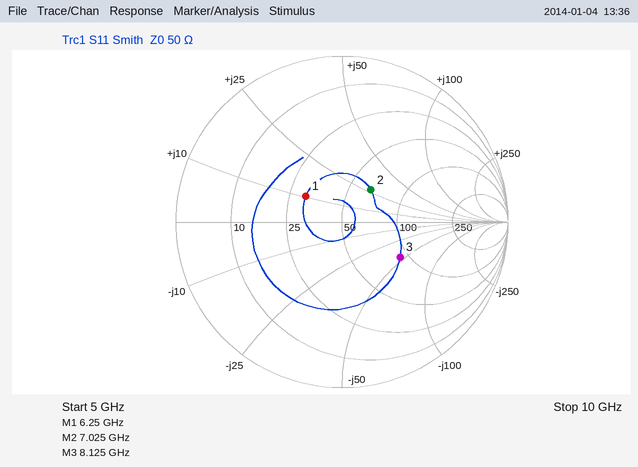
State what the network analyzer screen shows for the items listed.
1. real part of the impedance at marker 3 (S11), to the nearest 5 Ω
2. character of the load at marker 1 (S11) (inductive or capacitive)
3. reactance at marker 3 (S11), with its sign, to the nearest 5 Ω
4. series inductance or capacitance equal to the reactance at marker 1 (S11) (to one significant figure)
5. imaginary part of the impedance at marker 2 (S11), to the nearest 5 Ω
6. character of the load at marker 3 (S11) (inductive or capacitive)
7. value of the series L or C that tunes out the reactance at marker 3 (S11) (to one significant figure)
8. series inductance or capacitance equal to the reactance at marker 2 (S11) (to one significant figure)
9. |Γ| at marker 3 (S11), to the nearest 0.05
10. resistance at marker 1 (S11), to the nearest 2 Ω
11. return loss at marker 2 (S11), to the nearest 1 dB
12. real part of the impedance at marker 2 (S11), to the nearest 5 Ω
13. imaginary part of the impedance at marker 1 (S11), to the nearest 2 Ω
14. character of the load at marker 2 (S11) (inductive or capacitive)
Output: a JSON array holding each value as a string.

["90 Ω", "inductive", "-45 Ω", "300 pH", "+25 Ω", "capacitive", "900 pH", "600 pH", "0.40", "30 Ω", "12 dB", "65 Ω", "+10 Ω", "inductive"]
